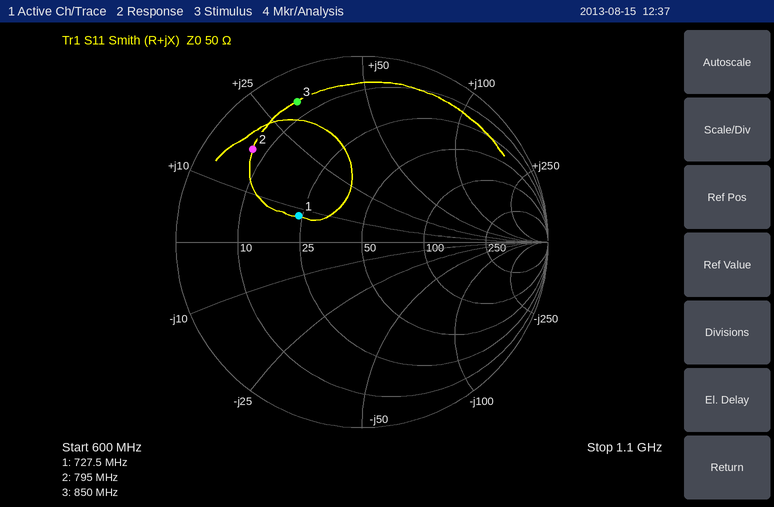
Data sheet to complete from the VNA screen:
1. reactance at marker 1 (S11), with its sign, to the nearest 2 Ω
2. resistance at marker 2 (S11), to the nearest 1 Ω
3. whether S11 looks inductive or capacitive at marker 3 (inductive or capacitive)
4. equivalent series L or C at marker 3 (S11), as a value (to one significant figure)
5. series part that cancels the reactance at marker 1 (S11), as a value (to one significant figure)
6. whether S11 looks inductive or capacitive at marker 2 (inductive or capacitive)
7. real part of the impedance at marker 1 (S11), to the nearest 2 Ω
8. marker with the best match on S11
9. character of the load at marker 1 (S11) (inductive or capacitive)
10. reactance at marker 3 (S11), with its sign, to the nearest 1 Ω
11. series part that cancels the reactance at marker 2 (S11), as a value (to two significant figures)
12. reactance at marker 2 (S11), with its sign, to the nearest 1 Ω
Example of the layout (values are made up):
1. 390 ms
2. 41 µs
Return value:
1. +8 Ω
2. 7 Ω
3. inductive
4. 6 nH
5. 30 pF
6. inductive
7. 24 Ω
8. marker 1
9. inductive
10. +32 Ω
11. 11 pF
12. +18 Ω
